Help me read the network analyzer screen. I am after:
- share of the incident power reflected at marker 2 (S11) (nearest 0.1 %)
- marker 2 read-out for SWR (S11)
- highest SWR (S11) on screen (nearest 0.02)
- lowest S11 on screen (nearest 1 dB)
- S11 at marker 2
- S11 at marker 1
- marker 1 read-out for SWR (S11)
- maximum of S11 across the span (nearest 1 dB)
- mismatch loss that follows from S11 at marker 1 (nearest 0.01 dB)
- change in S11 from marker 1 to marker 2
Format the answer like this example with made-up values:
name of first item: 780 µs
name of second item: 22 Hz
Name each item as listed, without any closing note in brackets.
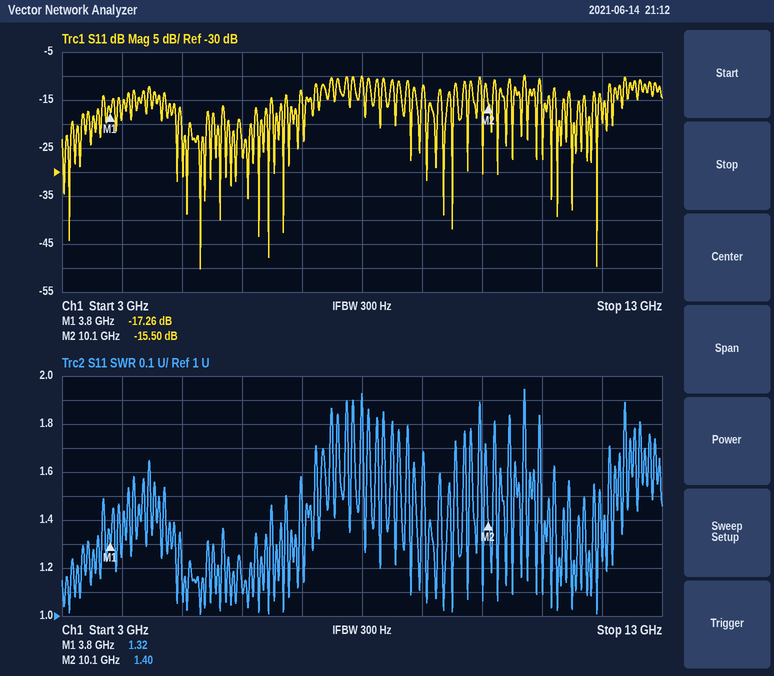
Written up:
share of the incident power reflected at marker 2 (S11): 2.8 %
marker 2 read-out for SWR: 1.40
highest SWR (S11) on screen: 1.94
lowest S11 on screen: -50 dB
S11 at marker 2: -15.50 dB
S11 at marker 1: -17.26 dB
marker 1 read-out for SWR: 1.32
maximum of S11 across the span: -10 dB
mismatch loss that follows from S11 at marker 1: 0.08 dB
change in S11 from marker 1 to marker 2: 1.76 dB
